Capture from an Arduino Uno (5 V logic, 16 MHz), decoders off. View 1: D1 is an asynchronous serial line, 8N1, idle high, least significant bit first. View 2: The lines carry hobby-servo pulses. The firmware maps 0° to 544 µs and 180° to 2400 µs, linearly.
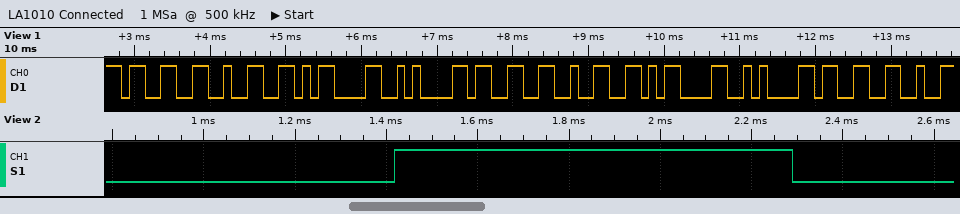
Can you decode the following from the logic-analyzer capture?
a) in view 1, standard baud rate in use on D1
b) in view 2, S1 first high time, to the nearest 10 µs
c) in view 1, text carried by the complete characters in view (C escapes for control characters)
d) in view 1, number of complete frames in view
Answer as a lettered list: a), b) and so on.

a) 9600 baud
b) 870 µs
c) "32\r\n32\r\n3"
d) 9
